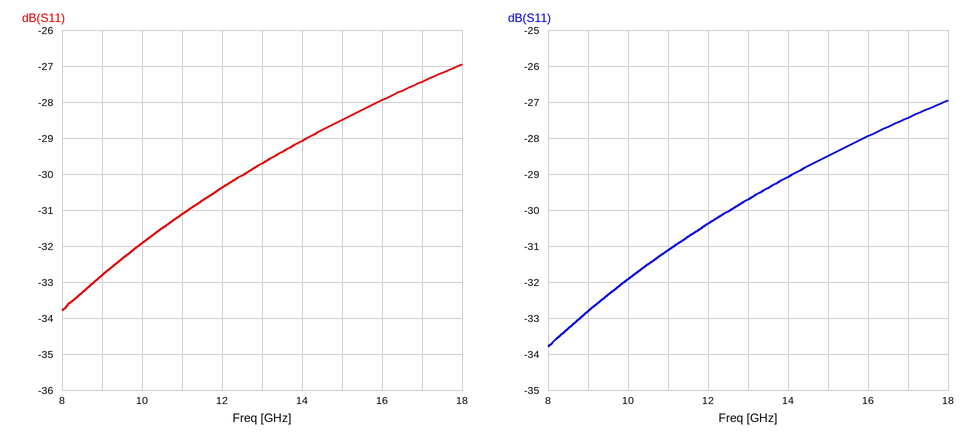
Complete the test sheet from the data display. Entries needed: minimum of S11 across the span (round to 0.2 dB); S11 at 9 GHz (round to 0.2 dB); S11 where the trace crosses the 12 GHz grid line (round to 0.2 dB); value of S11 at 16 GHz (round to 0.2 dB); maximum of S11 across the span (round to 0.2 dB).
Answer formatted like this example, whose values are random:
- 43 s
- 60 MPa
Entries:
- -33.8 dB
- -32.8 dB
- -30.4 dB
- -28.0 dB
- -27.0 dB
